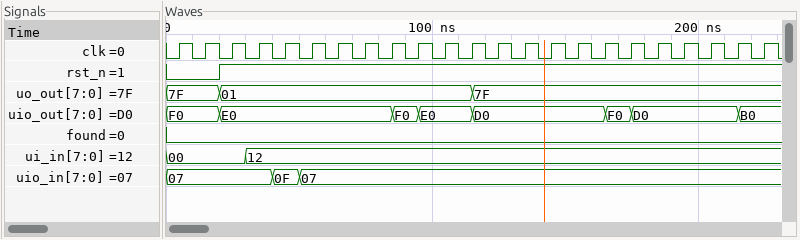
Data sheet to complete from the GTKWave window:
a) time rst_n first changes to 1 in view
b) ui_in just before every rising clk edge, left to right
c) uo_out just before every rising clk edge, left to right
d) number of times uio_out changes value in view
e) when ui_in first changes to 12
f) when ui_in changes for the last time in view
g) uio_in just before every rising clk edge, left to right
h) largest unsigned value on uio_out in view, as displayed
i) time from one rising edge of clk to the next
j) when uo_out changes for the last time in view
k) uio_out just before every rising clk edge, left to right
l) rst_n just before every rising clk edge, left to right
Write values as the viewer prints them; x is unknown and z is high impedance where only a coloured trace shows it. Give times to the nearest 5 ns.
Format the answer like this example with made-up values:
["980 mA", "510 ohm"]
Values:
["20 ns", "00, 00, 00, 12, 12, 12, 12, 12, 12, 12, 12, 12, 12, 12, 12, 12, 12, 12, 12, 12, 12, 12, 12", "7F, 7F, 01, 01, 01, 01, 01, 01, 01, 01, 01, 01, 7F, 7F, 7F, 7F, 7F, 7F, 7F, 7F, 7F, 7F, 7F", "7", "30 ns", "30 ns", "07, 07, 07, 07, 0F, 07, 07, 07, 07, 07, 07, 07, 07, 07, 07, 07, 07, 07, 07, 07, 07, 07, 07", "F0", "10 ns", "115 ns", "F0, F0, E0, E0, E0, E0, E0, E0, E0, F0, E0, E0, D0, D0, D0, D0, D0, F0, D0, D0, D0, D0, B0", "0 0 1 1 1 1 1 1 1 1 1 1 1 1 1 1 1 1 1 1 1 1 1"]
